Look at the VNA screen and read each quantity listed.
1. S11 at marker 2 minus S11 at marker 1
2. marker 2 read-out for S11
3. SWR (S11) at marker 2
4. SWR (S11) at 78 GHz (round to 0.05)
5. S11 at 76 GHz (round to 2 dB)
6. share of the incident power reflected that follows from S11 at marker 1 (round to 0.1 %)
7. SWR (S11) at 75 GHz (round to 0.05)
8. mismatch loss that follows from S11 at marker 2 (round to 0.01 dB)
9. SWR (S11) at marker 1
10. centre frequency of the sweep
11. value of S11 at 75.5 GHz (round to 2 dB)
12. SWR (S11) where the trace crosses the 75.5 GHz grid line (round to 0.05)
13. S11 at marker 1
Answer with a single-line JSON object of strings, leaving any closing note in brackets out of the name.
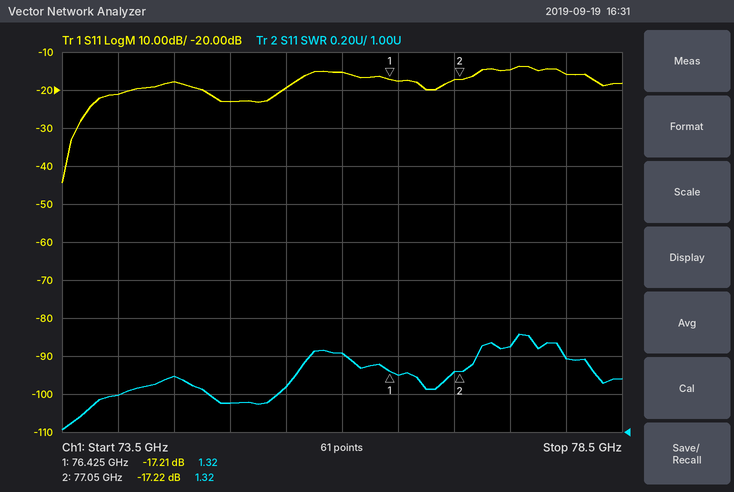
{"S11 at marker 2 minus S11 at marker 1": "-0.01 dB", "marker 2 read-out for S11": "-17.22 dB", "SWR (S11) at marker 2": "1.32", "SWR (S11) at 78 GHz": "1.40", "S11 at 76 GHz": "-16 dB", "share of the incident power reflected that follows from S11 at marker 1": "1.9 %", "SWR (S11) at 75 GHz": "1.15", "mismatch loss that follows from S11 at marker 2": "0.08 dB", "SWR (S11) at marker 1": "1.32", "centre frequency of the sweep": "76 GHz", "value of S11 at 75.5 GHz": "-20 dB", "SWR (S11) where the trace crosses the 75.5 GHz grid line": "1.25", "S11 at marker 1": "-17.21 dB"}
